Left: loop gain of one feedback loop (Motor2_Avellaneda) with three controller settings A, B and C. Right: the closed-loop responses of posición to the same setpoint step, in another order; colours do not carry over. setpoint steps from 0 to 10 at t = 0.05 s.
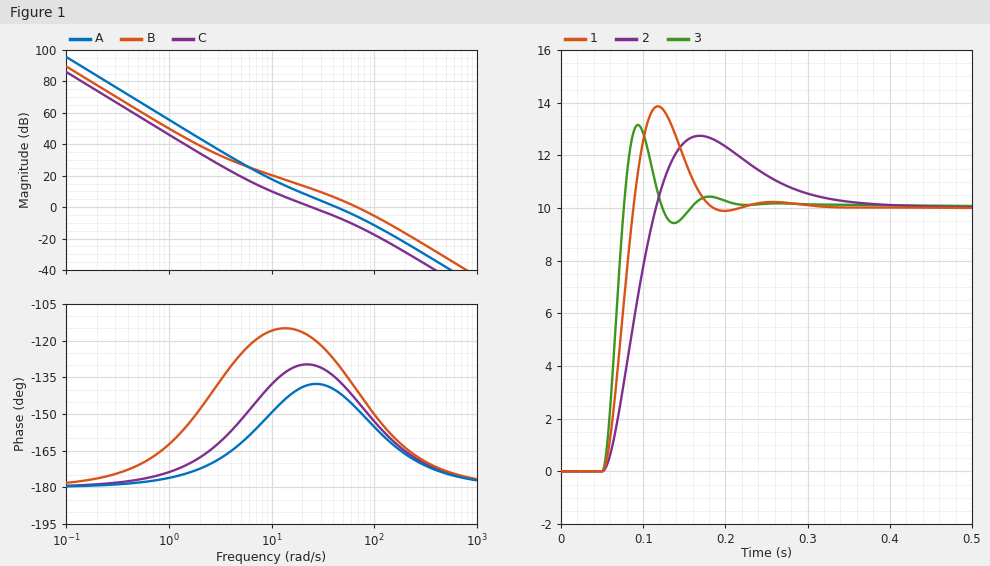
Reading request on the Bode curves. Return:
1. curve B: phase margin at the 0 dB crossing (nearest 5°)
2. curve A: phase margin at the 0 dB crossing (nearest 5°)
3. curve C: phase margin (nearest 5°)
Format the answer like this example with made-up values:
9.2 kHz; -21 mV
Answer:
40°; 40°; 50°
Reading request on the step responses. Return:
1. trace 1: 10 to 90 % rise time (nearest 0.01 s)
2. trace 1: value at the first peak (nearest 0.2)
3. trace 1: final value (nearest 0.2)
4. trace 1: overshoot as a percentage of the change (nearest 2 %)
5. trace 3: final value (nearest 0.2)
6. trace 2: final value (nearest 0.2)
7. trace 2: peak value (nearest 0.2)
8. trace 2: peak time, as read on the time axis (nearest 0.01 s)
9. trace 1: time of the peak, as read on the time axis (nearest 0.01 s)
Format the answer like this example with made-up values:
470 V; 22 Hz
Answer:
0.03 s; 13.8; 10.0; 38 %; 10.0; 10.0; 12.8; 0.17 s; 0.12 s
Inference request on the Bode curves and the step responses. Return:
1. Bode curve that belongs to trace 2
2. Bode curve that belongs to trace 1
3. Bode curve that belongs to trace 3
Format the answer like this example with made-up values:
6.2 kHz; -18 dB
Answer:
C; A; B
